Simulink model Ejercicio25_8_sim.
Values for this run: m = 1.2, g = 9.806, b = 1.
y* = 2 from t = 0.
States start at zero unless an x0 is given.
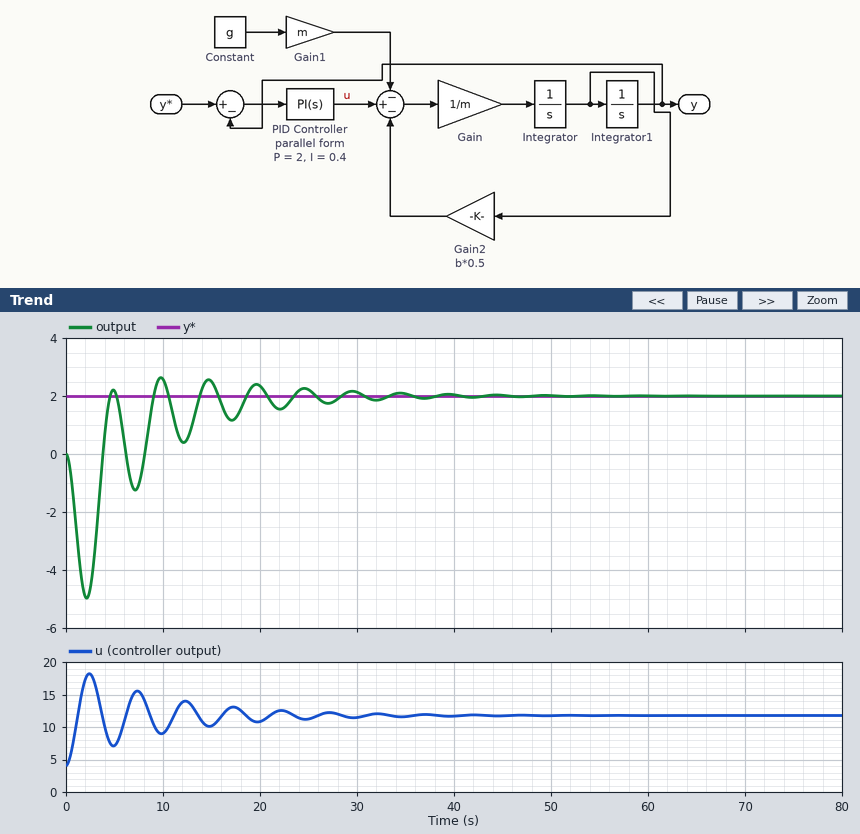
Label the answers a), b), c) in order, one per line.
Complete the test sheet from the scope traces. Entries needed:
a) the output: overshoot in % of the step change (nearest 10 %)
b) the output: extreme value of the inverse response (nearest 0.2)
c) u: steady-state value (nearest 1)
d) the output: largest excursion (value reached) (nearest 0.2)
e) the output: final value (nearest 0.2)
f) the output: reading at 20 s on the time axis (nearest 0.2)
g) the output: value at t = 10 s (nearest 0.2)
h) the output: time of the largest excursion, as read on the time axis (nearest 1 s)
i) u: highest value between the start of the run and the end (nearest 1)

a) 30 %
b) -5.0
c) 12
d) 2.6
e) 2.0
f) 2.4
g) 2.6
h) 10 s
i) 18
